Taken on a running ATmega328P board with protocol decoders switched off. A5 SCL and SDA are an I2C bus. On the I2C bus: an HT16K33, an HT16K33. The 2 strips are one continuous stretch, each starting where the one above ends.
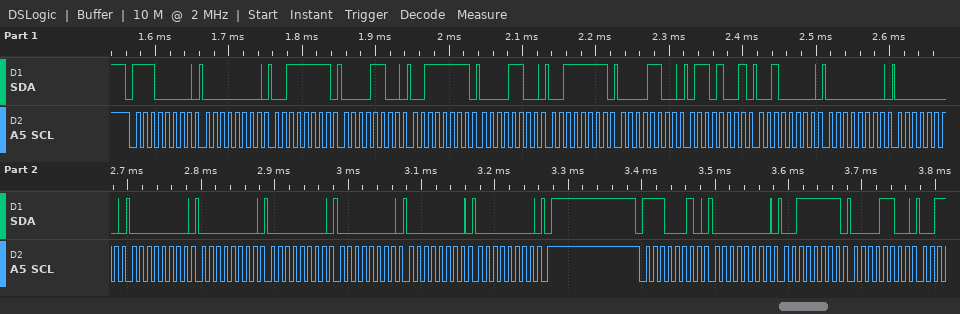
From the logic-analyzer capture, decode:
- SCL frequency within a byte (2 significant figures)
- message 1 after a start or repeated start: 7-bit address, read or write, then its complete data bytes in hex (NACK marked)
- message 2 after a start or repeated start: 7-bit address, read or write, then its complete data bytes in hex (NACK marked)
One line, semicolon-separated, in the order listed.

100 kHz; 0x70 write: 00 3F 0C 3F 0C 3F 0C 69 20 00 00 00 00 00 00 00 00; 0x71 write: 00 3F 0C
